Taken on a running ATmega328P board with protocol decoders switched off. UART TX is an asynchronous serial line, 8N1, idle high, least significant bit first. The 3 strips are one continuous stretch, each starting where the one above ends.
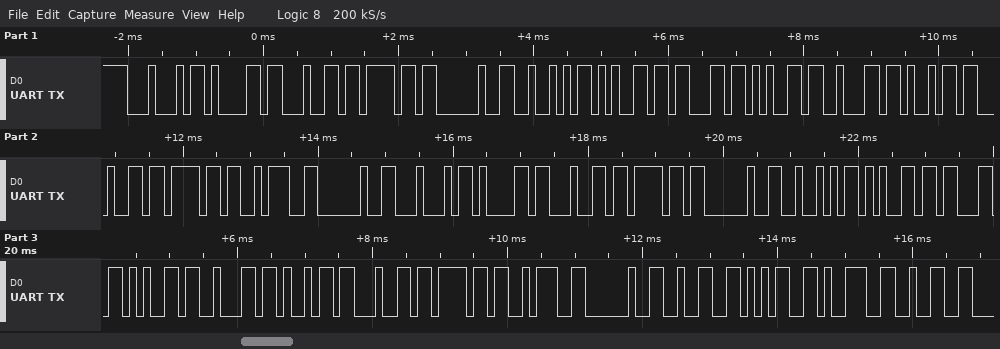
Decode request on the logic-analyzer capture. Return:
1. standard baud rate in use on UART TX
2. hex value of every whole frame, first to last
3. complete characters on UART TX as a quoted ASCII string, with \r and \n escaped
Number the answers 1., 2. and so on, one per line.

1. 9600 baud
2. 44 61 64 6F 20 52 65 63 65 62 69 64 6F 3A 20 44 61 64 6F 20 52 65 63 65 62 69 64 6F 3A 20 32 35 39 32
3. "Dado Recebido: Dado Recebido: 2592"
